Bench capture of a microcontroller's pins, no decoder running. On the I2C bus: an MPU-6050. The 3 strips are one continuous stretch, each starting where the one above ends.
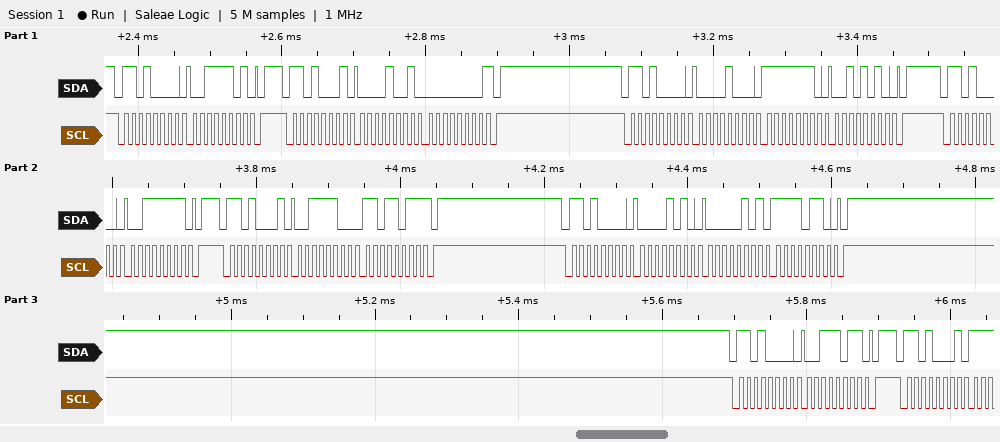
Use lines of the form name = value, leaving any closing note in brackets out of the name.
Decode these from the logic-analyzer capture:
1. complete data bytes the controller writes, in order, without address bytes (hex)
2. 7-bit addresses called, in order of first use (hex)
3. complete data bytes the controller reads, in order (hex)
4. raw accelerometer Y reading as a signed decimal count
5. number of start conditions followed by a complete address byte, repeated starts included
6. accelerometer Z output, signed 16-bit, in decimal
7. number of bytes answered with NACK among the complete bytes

complete data bytes the controller writes, in order, without address bytes = 3D 08 FE 2A 3F 0A 05 F6 3B
7-bit addresses called, in order of first use = 0x68
complete data bytes the controller reads, in order = 09 00 3C DB
raw accelerometer Y reading as a signed decimal count = 2304
number of start conditions followed by a complete address byte, repeated starts included = 8
accelerometer Z output, signed 16-bit, in decimal = 15579
number of bytes answered with NACK among the complete bytes = 2
